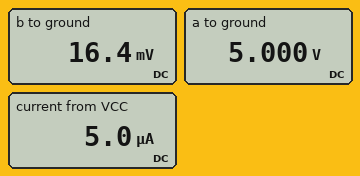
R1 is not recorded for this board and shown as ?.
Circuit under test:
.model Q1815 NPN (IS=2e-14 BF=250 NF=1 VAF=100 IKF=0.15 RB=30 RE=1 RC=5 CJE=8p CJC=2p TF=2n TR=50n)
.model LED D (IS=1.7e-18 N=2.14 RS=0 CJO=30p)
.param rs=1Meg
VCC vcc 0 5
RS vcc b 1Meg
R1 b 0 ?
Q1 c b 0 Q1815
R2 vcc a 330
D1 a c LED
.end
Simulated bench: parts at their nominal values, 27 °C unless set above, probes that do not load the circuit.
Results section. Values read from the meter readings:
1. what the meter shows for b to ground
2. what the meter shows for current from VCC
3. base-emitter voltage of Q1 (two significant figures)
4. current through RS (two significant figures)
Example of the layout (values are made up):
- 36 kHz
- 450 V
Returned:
- 16.4 mV
- 5.0 µA
- 16 mV
- 5.0 µA
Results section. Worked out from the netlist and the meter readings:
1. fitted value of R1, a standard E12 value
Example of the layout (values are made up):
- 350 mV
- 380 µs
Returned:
- 3.3 kΩ
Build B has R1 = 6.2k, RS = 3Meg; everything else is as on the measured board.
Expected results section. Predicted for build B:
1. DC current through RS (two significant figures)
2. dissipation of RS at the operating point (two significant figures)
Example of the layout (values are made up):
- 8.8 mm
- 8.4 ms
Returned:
- 1.7 µA
- 8.3 µW
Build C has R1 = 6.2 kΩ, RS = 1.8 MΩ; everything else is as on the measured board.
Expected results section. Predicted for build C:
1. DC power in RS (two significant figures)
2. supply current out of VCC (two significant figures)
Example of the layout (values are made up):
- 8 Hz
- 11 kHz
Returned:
- 14 µW
- 2.8 µA
